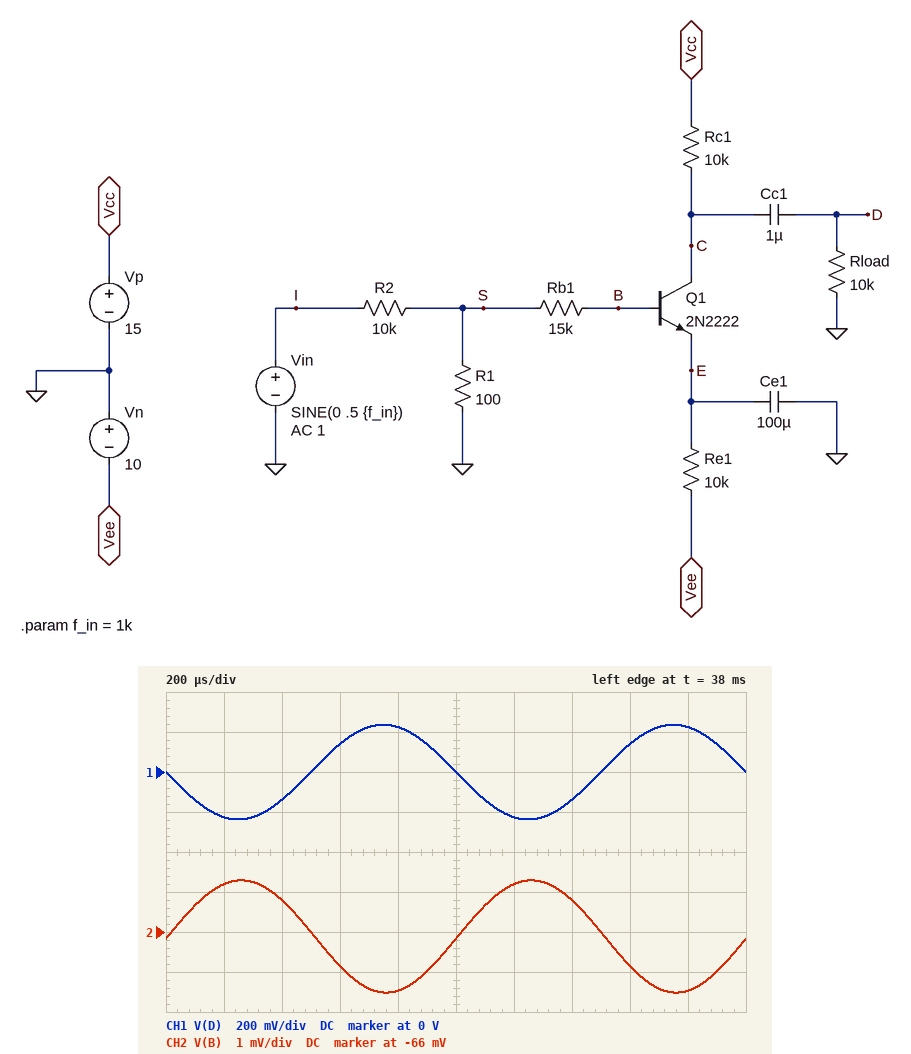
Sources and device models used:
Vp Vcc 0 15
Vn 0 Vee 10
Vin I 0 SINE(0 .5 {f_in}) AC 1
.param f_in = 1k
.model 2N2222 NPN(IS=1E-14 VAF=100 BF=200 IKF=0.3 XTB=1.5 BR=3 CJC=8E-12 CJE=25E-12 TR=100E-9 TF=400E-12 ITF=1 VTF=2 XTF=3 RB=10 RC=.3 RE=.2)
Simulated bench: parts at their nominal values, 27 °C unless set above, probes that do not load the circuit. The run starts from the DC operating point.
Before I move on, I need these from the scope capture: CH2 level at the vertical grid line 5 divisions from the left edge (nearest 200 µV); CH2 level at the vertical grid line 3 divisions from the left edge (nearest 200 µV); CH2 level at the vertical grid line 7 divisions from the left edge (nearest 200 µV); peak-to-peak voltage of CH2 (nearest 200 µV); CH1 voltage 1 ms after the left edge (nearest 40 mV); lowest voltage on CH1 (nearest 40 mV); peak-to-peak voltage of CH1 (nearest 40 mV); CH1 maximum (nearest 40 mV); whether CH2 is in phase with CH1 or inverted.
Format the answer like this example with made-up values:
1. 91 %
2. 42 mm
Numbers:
1. -66.2 mV
2. -66.8 mV
3. -65.2 mV
4. 2.8 mV
5. 0 V
6. -240 mV
7. 480 mV
8. 240 mV
9. inverted
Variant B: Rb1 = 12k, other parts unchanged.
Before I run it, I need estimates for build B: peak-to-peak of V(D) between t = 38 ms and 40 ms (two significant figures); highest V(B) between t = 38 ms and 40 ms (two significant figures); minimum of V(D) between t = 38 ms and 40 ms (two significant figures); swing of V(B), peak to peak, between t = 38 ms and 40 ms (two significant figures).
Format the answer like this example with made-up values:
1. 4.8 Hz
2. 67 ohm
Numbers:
1. 550 mV
2. -51 mV
3. -280 mV
4. 3.3 mV
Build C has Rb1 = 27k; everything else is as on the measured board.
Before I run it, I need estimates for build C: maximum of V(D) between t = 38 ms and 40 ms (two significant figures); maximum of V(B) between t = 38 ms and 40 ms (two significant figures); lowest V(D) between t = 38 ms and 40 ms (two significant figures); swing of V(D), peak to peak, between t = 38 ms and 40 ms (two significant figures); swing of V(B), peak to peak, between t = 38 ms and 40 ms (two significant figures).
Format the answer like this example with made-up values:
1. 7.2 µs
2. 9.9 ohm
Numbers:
1. 150 mV
2. -120 mV
3. -150 mV
4. 300 mV
5. 1.8 mV
